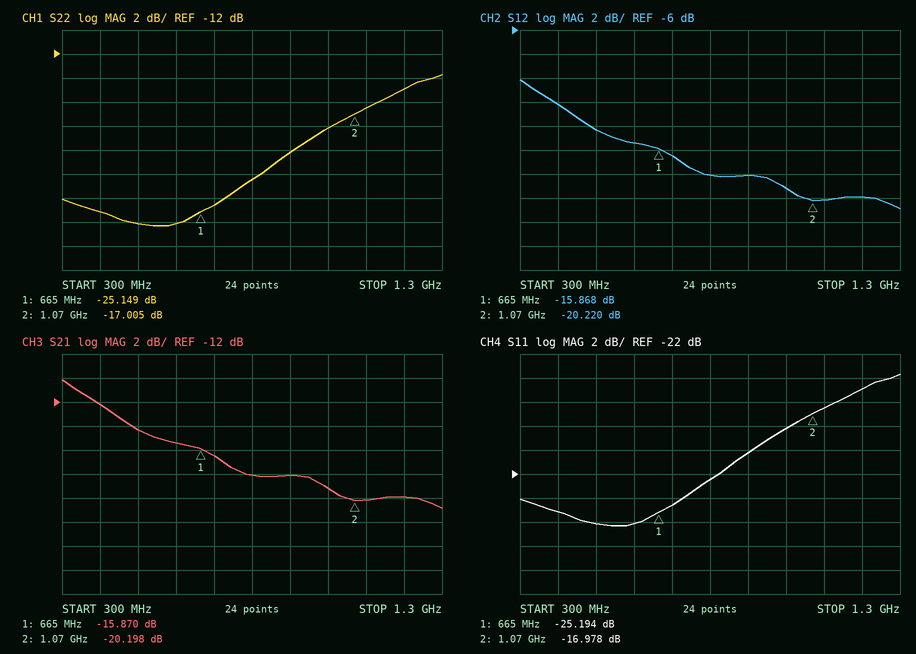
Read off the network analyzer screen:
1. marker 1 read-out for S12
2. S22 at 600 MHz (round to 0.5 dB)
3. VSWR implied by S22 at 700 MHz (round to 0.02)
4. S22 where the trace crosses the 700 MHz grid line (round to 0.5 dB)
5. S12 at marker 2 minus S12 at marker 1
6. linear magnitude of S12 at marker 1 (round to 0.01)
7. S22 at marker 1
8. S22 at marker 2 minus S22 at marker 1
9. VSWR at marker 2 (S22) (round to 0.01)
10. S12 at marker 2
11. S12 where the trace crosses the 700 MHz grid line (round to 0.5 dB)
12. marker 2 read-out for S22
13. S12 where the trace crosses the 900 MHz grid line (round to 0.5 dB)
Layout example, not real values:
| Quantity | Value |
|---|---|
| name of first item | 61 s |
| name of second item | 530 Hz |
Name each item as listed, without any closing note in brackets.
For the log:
| Quantity | Value |
|---|---|
| marker 1 read-out for S12 | -15.868 dB |
| S22 at 600 MHz | -26.0 dB |
| VSWR implied by S22 at 700 MHz | 1.12 |
| S22 where the trace crosses the 700 MHz grid line | -24.5 dB |
| S12 at marker 2 minus S12 at marker 1 | -4.352 dB |
| linear magnitude of S12 at marker 1 | 0.16 |
| S22 at marker 1 | -25.149 dB |
| S22 at marker 2 minus S22 at marker 1 | 8.144 dB |
| VSWR at marker 2 (S22) | 1.33 |
| S12 at marker 2 | -20.220 dB |
| S12 where the trace crosses the 700 MHz grid line | -16.5 dB |
| marker 2 read-out for S22 | -17.005 dB |
| S12 where the trace crosses the 900 MHz grid line | -18.0 dB |
